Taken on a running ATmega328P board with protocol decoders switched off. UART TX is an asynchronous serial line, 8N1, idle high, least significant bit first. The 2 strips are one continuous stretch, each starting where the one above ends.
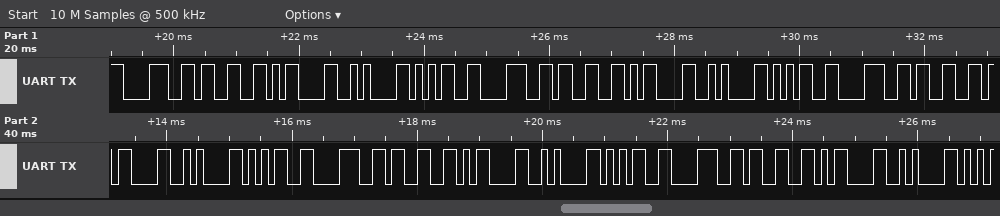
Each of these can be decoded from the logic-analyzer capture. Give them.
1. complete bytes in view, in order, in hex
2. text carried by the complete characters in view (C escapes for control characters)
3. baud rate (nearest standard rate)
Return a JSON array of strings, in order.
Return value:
["0x38 0x33 0x0D 0x0A 0x35 0x38 0x33 0x0D 0x0A 0x35 0x38 0x33 0x0D 0x0A 0x35 0x38 0x33 0x0D 0x0A 0x35 0x38 0x33 0x0D 0x0A", "\"83\\r\\n583\\r\\n583\\r\\n583\\r\\n583\\r\\n\"", "9600 baud"]
